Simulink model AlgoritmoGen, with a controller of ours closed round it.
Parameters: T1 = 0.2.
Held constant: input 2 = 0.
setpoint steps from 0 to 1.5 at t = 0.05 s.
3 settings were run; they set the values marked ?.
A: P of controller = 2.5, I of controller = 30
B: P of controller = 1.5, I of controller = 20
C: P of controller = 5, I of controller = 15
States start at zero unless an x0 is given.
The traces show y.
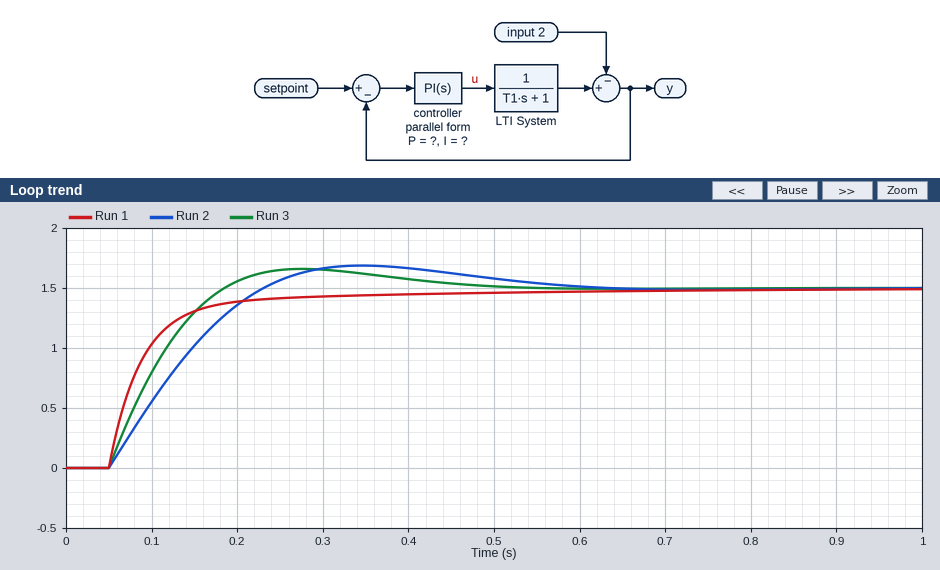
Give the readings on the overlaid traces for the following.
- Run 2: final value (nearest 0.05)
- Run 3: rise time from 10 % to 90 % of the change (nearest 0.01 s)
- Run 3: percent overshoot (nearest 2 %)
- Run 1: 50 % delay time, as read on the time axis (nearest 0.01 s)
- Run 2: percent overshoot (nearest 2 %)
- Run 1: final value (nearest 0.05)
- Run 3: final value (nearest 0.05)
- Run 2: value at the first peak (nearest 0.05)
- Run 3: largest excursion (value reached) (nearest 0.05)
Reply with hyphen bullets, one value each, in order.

- 1.50
- 0.10 s
- 10 %
- 0.08 s
- 12 %
- 1.50
- 1.50
- 1.70
- 1.65
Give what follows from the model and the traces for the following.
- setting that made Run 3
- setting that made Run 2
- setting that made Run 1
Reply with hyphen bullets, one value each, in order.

- A
- B
- C
